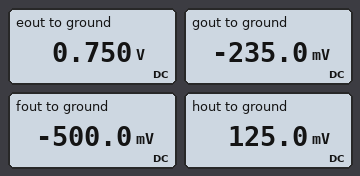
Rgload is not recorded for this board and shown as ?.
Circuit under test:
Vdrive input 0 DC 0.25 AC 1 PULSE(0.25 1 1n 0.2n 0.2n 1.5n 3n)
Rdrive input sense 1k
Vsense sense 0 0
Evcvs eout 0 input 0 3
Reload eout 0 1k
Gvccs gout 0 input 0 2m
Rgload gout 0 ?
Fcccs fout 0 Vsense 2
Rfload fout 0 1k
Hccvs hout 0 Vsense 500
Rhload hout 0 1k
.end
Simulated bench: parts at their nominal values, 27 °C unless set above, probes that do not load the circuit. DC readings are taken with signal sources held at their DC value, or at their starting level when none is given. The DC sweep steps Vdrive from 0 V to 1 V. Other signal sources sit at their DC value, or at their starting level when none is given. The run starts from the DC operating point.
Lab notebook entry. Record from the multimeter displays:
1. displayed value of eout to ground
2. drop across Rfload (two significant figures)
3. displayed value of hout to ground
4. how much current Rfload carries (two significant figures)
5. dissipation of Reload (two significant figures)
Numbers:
0.750 V
500 mV
125.0 mV
500 µA
560 µW
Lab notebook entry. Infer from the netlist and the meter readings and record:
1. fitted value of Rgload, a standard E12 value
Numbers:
470 Ω
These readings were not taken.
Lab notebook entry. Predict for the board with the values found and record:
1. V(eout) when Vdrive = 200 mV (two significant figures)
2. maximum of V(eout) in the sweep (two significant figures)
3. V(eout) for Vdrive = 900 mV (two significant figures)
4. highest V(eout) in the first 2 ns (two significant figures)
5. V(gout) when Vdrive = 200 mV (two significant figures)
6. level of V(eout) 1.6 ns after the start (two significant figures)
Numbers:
600 mV
3.0 V
2.7 V
3.0 V
-190 mV
3.0 V
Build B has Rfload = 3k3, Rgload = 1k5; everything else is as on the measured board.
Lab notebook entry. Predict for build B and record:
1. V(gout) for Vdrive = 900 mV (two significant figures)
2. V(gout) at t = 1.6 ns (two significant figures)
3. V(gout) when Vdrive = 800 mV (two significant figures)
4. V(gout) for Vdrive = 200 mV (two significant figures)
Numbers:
-2.7 V
-3.0 V
-2.4 V
-600 mV
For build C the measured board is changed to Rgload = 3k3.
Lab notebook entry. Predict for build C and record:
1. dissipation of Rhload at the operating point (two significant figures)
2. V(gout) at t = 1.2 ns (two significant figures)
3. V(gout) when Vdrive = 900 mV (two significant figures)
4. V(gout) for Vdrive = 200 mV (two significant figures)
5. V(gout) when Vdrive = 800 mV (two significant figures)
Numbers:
16 µW
-6.6 V
-5.9 V
-1.3 V
-5.3 V
